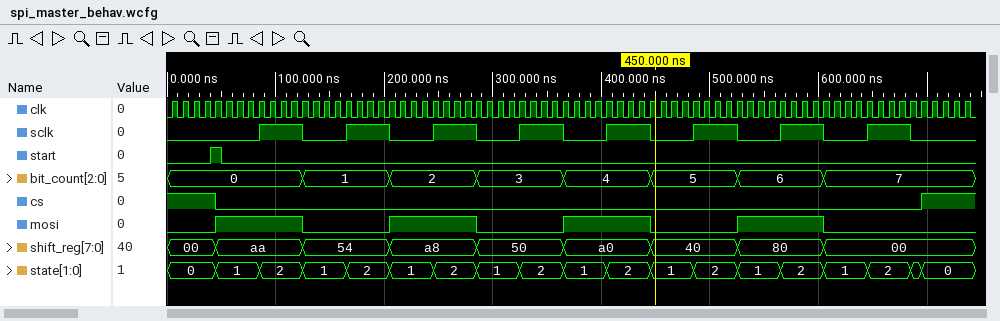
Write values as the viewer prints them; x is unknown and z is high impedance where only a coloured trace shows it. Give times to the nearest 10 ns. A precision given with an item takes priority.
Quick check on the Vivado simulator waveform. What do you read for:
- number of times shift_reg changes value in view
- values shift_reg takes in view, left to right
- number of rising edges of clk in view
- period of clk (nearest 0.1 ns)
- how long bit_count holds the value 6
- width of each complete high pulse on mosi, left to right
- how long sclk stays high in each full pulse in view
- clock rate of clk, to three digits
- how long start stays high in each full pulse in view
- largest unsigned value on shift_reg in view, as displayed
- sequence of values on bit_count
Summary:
8
00, aa, 54, a8, 50, a0, 40, 80, 00
74
10 ns
80 ns
80 ns, 80 ns, 80 ns, 80 ns
40 ns, 40 ns, 40 ns, 40 ns, 40 ns, 40 ns, 40 ns, 40 ns
100 MHz
10 ns
aa
0, 1, 2, 3, 4, 5, 6, 7
